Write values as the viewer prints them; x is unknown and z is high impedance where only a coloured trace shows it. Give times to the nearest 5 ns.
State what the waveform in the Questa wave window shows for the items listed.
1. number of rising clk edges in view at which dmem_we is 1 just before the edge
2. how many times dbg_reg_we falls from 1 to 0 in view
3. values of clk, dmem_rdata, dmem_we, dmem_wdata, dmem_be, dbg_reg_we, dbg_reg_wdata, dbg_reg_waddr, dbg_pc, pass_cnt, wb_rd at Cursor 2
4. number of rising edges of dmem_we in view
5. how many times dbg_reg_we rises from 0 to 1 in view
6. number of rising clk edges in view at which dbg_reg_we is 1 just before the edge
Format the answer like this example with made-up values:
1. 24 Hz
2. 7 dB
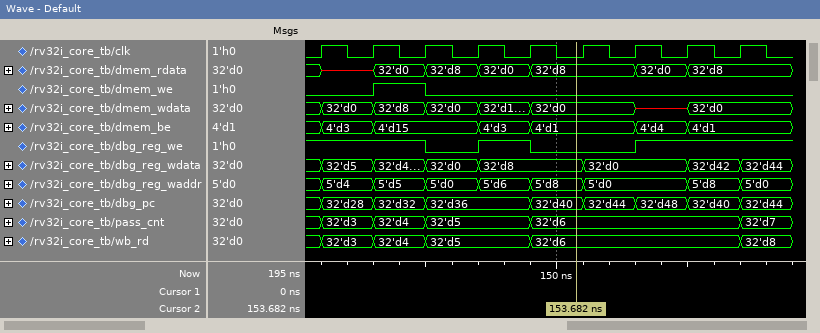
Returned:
1. 1
2. 2
3. clk=0, dmem_rdata=32'd8, dmem_we=0, dmem_wdata=32'd0, dmem_be=4'd1, dbg_reg_we=0, dbg_reg_wdata=32'd8, dbg_reg_waddr=5'd8, dbg_pc=32'd40, pass_cnt=32'd6, wb_rd=32'd6
4. 1
5. 2
6. 6
